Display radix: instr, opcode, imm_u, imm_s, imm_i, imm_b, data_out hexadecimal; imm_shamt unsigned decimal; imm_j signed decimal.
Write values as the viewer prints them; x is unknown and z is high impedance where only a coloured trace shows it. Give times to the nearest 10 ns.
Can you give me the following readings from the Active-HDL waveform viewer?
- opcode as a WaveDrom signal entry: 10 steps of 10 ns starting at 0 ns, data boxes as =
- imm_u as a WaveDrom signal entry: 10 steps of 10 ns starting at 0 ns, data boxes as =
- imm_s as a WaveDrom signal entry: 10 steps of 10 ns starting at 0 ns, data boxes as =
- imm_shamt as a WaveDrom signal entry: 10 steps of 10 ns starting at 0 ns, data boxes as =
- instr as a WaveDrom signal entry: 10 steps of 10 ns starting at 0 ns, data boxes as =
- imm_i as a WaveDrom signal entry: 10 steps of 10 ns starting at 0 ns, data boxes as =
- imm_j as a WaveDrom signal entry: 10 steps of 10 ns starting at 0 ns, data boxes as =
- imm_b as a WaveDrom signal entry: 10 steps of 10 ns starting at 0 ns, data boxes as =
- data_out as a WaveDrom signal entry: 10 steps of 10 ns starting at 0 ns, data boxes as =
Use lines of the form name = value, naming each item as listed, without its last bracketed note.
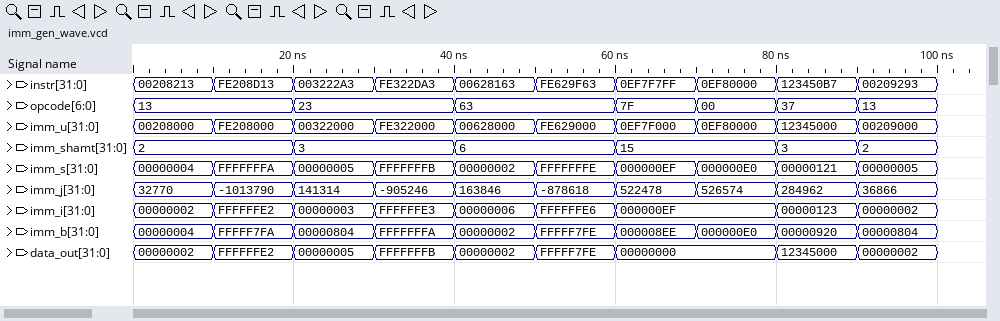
opcode as a WaveDrom signal entry: 10 steps of 10 ns starting at 0 ns, data boxes as = = {name: 'opcode', wave: '=.=.=.====', data: '13 23 63 7F 00 37 13'}
imm_u as a WaveDrom signal entry: 10 steps of 10 ns starting at 0 ns, data boxes as = = {name: 'imm_u', wave: '==========', data: '00208000 FE208000 00322000 FE322000 00628000 FE629000 0EF7F000 0EF80000 12345000 00209000'}
imm_s as a WaveDrom signal entry: 10 steps of 10 ns starting at 0 ns, data boxes as = = {name: 'imm_s', wave: '==========', data: '00000004 FFFFFFFA 00000005 FFFFFFFB 00000002 FFFFFFFE 000000EF 000000E0 00000121 00000005'}
imm_shamt as a WaveDrom signal entry: 10 steps of 10 ns starting at 0 ns, data boxes as = = {name: 'imm_shamt', wave: '=.=.=.=.==', data: '2 3 6 15 3 2'}
instr as a WaveDrom signal entry: 10 steps of 10 ns starting at 0 ns, data boxes as = = {name: 'instr', wave: '==========', data: '00208213 FE208D13 003222A3 FE322DA3 00628163 FE629F63 0EF7F7FF 0EF80000 123450B7 00209293'}
imm_i as a WaveDrom signal entry: 10 steps of 10 ns starting at 0 ns, data boxes as = = {name: 'imm_i', wave: '=======.==', data: '00000002 FFFFFFE2 00000003 FFFFFFE3 00000006 FFFFFFE6 000000EF 00000123 00000002'}
imm_j as a WaveDrom signal entry: 10 steps of 10 ns starting at 0 ns, data boxes as = = {name: 'imm_j', wave: '==========', data: '32770 -1013790 141314 -905246 163846 -878618 522478 526574 284962 36866'}
imm_b as a WaveDrom signal entry: 10 steps of 10 ns starting at 0 ns, data boxes as = = {name: 'imm_b', wave: '==========', data: '00000004 FFFFF7FA 00000804 FFFFFFFA 00000002 FFFFF7FE 000008EE 000000E0 00000920 00000804'}
data_out as a WaveDrom signal entry: 10 steps of 10 ns starting at 0 ns, data boxes as = = {name: 'data_out', wave: '=======.==', data: '00000002 FFFFFFE2 00000005 FFFFFFFB 00000002 FFFFF7FE 00000000 12345000 00000002'}
